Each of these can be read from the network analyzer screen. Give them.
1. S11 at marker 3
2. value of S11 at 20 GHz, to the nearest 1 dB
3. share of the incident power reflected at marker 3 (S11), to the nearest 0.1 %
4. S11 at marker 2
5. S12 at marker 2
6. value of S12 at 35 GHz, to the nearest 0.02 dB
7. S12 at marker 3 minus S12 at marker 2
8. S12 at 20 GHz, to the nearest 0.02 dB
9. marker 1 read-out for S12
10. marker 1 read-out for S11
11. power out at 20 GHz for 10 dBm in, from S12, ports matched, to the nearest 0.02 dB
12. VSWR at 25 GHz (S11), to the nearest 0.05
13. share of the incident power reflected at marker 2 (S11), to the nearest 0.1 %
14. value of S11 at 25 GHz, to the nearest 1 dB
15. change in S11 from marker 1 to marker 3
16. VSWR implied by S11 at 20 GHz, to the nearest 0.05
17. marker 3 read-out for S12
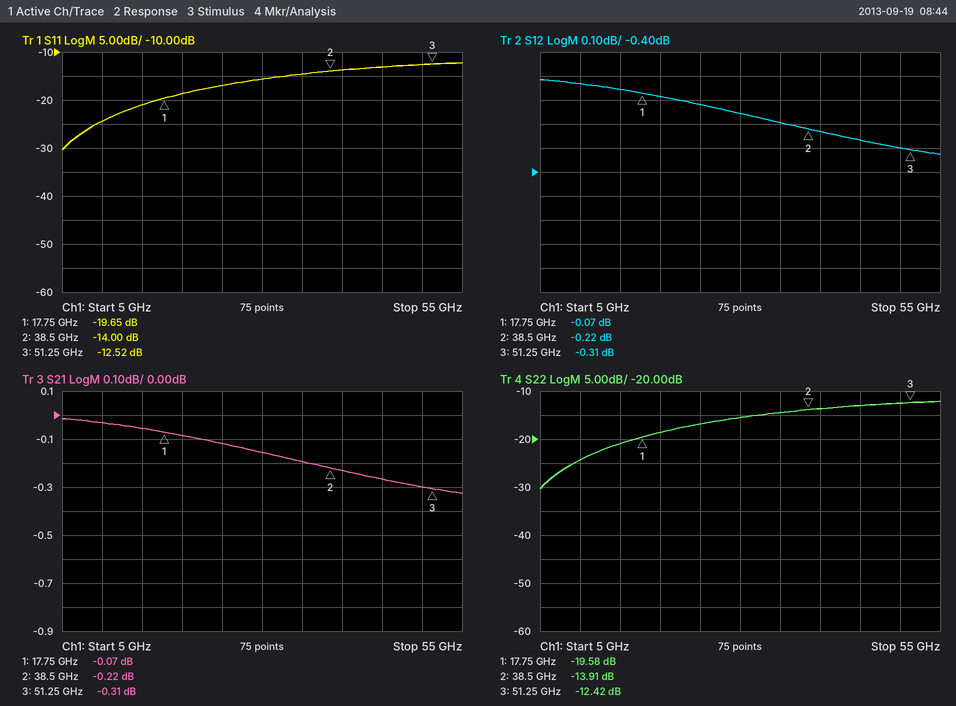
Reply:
-12.52 dB
-19 dB
5.6 %
-14.00 dB
-0.22 dB
-0.20 dB
-0.09 dB
-0.08 dB
-0.07 dB
-19.65 dB
9.92 dBm
1.35
4.0 %
-17 dB
7.13 dB
1.25
-0.31 dB
